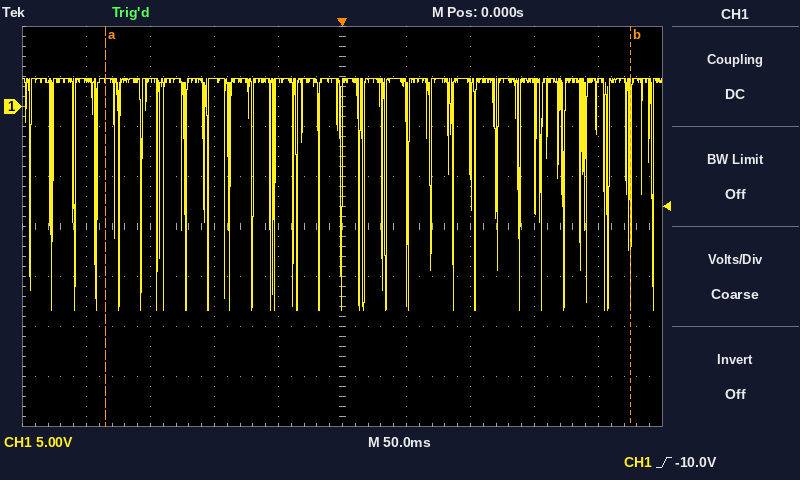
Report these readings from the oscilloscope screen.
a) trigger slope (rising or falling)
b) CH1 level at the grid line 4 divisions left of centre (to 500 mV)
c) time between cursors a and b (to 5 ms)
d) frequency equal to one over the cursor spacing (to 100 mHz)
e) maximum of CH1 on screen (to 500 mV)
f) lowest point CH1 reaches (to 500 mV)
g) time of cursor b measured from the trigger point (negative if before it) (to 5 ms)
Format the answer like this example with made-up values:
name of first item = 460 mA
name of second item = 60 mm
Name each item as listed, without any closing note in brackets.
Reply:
trigger slope = rising
CH1 level at the grid line 4 divisions left of centre = 2.5 V
time between cursors a and b = 410 ms
frequency equal to one over the cursor spacing = 2.4 Hz
maximum of CH1 on screen = 3.0 V
lowest point CH1 reaches = -20.5 V
time of cursor b measured from the trigger point (negative if before it) = +225 ms
